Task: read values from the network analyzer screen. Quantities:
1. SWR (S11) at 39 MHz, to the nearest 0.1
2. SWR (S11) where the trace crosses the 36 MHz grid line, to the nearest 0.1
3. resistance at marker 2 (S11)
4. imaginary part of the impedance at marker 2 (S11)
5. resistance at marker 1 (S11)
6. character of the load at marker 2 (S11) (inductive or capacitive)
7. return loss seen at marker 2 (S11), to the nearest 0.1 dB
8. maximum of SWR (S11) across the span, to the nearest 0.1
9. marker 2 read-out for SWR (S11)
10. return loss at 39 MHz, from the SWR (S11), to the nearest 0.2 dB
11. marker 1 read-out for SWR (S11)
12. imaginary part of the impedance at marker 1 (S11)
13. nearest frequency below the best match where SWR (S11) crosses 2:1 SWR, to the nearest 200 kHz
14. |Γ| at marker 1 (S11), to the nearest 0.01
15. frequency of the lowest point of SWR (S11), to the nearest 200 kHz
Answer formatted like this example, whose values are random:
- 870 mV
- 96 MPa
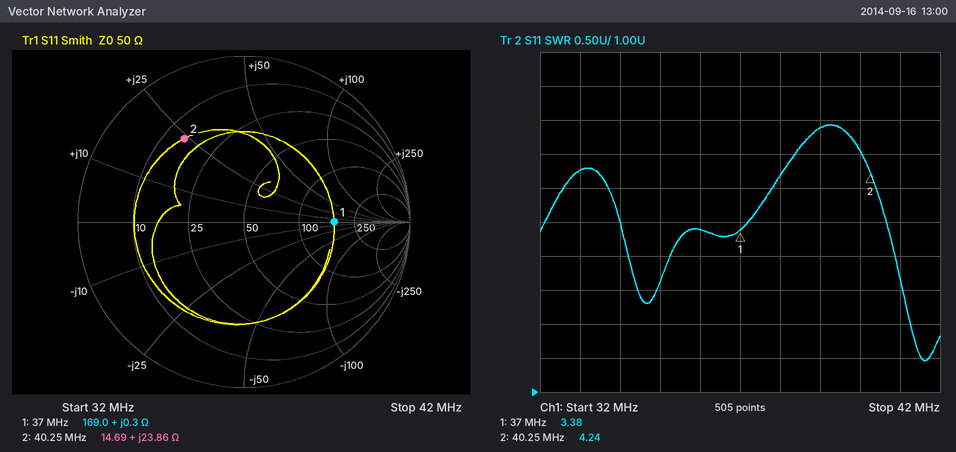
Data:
- 4.9
- 3.4
- 14.69 Ω
- +23.86 Ω
- 169.0 Ω
- inductive
- 4.2 dB
- 4.9
- 4.24
- 3.6 dB
- 3.38
- +0.3 Ω
- 41.2 MHz
- 0.54
- 41.6 MHz
